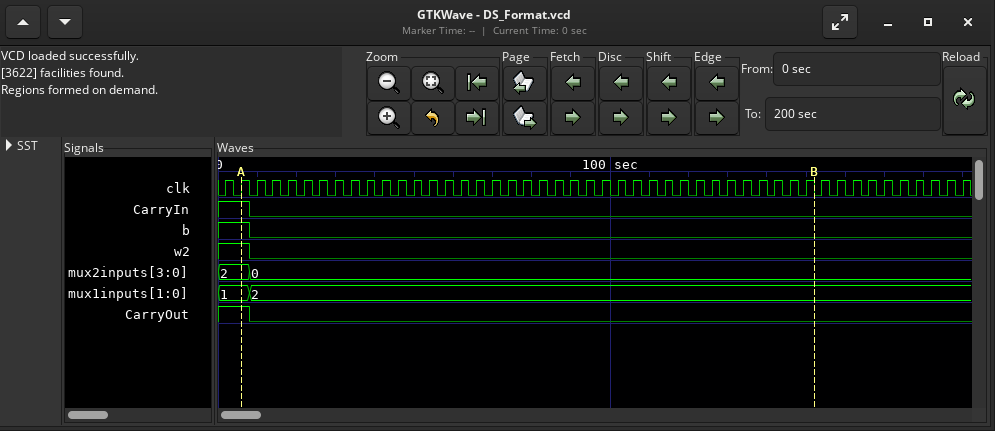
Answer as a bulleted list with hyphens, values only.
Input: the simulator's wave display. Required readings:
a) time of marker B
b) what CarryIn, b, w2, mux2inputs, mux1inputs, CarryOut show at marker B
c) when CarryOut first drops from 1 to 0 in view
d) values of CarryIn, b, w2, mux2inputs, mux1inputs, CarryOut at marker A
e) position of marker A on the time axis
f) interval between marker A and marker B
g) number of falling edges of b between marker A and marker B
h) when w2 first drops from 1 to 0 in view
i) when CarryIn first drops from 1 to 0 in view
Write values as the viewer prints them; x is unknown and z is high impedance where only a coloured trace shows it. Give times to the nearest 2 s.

- 152 s
- CarryIn=0, b=0, w2=0, mux2inputs=0, mux1inputs=2, CarryOut=0
- 8 s
- CarryIn=1, b=1, w2=1, mux2inputs=2, mux1inputs=1, CarryOut=1
- 6 s
- 146 s
- 1
- 8 s
- 8 s
